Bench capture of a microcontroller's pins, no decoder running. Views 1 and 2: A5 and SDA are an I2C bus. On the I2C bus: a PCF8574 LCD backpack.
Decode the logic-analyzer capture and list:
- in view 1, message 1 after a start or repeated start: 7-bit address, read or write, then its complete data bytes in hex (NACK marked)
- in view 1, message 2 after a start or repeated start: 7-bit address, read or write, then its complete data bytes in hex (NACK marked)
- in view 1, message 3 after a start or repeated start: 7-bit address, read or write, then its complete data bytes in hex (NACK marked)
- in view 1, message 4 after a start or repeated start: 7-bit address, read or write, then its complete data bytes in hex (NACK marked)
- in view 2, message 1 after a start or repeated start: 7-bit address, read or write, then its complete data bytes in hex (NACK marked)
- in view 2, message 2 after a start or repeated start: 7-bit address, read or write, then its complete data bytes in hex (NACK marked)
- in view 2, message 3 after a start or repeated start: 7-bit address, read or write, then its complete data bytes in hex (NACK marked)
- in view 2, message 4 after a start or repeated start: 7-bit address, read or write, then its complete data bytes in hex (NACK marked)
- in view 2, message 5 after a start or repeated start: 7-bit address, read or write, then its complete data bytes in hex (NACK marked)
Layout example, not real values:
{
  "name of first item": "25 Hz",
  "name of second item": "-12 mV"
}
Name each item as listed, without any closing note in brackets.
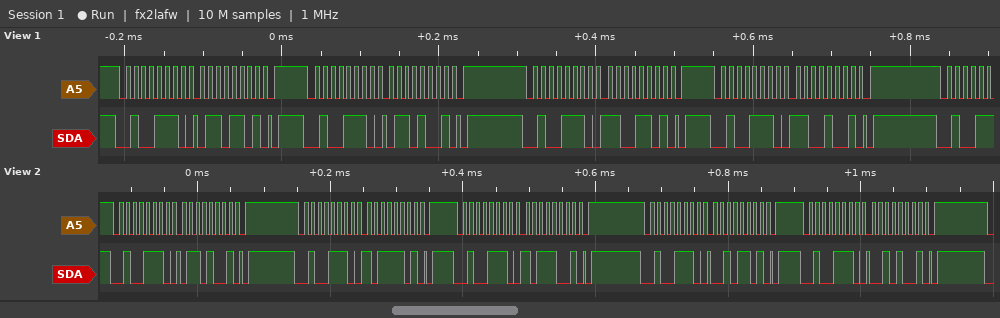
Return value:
{
  "in view 1, message 1 after a start or repeated start: 7-bit address, read or write, then its complete data bytes in hex": "0x27 write: 6D",
  "in view 1, message 2 after a start or repeated start: 7-bit address, read or write, then its complete data bytes in hex": "0x27 write: 69",
  "in view 1, message 3 after a start or repeated start: 7-bit address, read or write, then its complete data bytes in hex": "0x27 write: CD",
  "in view 1, message 4 after a start or repeated start: 7-bit address, read or write, then its complete data bytes in hex": "0x27 write: C9",
  "in view 2, message 1 after a start or repeated start: 7-bit address, read or write, then its complete data bytes in hex": "0x27 write: 69",
  "in view 2, message 2 after a start or repeated start: 7-bit address, read or write, then its complete data bytes in hex": "0x27 write: BD",
  "in view 2, message 3 after a start or repeated start: 7-bit address, read or write, then its complete data bytes in hex": "0x27 write: B9",
  "in view 2, message 4 after a start or repeated start: 7-bit address, read or write, then its complete data bytes in hex": "0x27 write: 2D",
  "in view 2, message 5 after a start or repeated start: 7-bit address, read or write, then its complete data bytes in hex": "0x27 write: 29"
}
